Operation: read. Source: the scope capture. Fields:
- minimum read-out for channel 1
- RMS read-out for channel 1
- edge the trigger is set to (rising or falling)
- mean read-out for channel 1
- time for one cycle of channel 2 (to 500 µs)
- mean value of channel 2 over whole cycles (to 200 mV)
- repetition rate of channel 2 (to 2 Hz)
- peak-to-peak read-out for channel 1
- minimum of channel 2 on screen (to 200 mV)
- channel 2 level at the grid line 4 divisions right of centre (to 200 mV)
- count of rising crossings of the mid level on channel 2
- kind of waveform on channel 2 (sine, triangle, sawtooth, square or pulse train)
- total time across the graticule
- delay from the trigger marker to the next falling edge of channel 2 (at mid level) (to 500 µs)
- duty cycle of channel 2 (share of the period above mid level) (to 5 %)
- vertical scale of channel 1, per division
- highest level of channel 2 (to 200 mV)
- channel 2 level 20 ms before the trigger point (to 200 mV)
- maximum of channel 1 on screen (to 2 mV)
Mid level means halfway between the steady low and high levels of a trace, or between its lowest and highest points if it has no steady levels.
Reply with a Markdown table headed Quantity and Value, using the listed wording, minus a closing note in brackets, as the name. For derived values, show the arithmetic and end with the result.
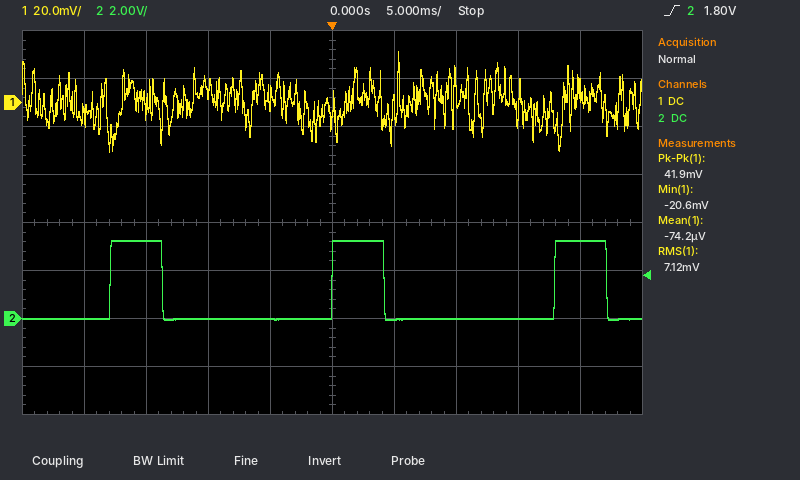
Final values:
| Quantity | Value |
|---|---|
| minimum read-out for channel 1 | -20.6 mV |
| RMS read-out for channel 1 | 7.12 mV |
| edge the trigger is set to | rising |
| mean read-out for channel 1 | -74.2 µV |
| time for one cycle of channel 2 | 18.0 ms |
| mean value of channel 2 over whole cycles | 0.0 V + 0.25 × (3.2 V − (0.0 V)) ≈ 800 mV |
| repetition rate of channel 2 | 1 / 18.0 ms ≈ 56 Hz |
| peak-to-peak read-out for channel 1 | 41.9 mV |
| minimum of channel 2 on screen | 0.0 V |
| channel 2 level at the grid line 4 divisions right of centre | 3.2 V |
| count of rising crossings of the mid level on channel 2 | 3 |
| kind of waveform on channel 2 | pulse train |
| total time across the graticule | 50 ms |
| delay from the trigger marker to the next falling edge of channel 2 (at mid level) | 4.0 ms |
| duty cycle of channel 2 (share of the period above mid level) | 25 % |
| vertical scale of channel 1, per division | 20 mV |
| highest level of channel 2 | 3.2 V |
| channel 2 level 20 ms before the trigger point | 0.0 V |
| maximum of channel 1 on screen | 22 mV |
